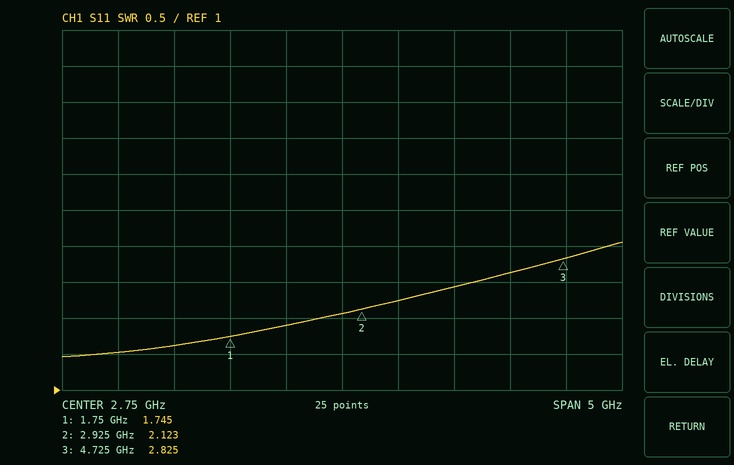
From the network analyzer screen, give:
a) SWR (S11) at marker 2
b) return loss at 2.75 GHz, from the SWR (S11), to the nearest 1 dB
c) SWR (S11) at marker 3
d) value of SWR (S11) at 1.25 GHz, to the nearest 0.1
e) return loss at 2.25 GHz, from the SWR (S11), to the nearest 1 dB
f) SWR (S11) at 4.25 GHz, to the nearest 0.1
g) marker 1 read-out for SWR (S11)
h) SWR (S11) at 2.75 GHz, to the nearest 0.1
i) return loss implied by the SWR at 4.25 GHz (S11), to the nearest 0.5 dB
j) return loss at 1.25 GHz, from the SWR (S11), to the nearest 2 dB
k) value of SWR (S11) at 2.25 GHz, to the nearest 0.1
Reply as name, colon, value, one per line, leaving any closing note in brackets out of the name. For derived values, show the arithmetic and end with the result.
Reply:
SWR (S11) at marker 2: 2.123
return loss at 2.75 GHz, from the SWR (S11), to the nearest 1 dB: −20 log10((2.1 − 1)/(2.1 + 1)) ≈ 9 dB
SWR (S11) at marker 3: 2.825
value of SWR (S11) at 1.25 GHz, to the nearest 0.1: 1.6
return loss at 2.25 GHz, from the SWR (S11), to the nearest 1 dB: −20 log10((1.9 − 1)/(1.9 + 1)) ≈ 10 dB
SWR (S11) at 4.25 GHz, to the nearest 0.1: 2.6
marker 1 read-out for SWR: 1.745
SWR (S11) at 2.75 GHz, to the nearest 0.1: 2.1
return loss implied by the SWR at 4.25 GHz (S11), to the nearest 0.5 dB: −20 log10((2.6 − 1)/(2.6 + 1)) ≈ 7.0 dB
return loss at 1.25 GHz, from the SWR (S11), to the nearest 2 dB: −20 log10((1.6 − 1)/(1.6 + 1)) ≈ 12.7 dB, so 12 dB to the nearest 2 dB
value of SWR (S11) at 2.25 GHz, to the nearest 0.1: 1.9
